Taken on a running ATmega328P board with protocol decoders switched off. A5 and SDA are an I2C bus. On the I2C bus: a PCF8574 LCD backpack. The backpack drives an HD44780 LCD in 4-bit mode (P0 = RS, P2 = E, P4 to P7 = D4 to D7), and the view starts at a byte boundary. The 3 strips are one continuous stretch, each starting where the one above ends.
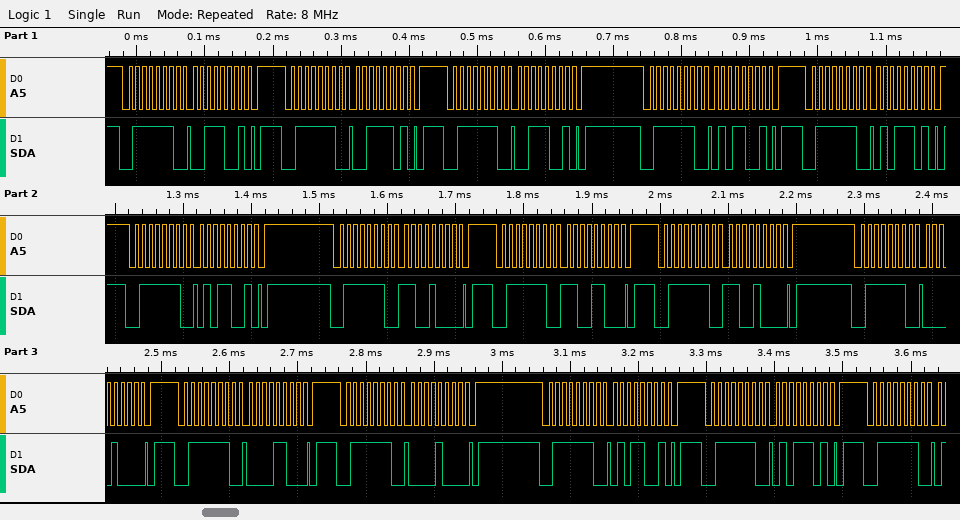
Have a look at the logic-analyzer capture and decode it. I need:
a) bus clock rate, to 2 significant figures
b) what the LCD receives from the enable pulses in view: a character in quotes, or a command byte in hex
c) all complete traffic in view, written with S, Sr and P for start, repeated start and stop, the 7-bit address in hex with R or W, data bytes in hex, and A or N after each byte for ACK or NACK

100 kHz
'5' 0xC0
S 3FW A 39 A P S 3FW A 3D A P S 3FW A 39 A P S 3FW A 59 A P S 3FW A 5D A P S 3FW A 59 A P S 3FW A C8 A P S 3FW A CC A P S 3FW A C8 A P S 3FW A 08 A P S 3FW A 0C A P S 3FW A 08 A P S 3FW A 59 A P S 3FW A 5D A P S 3FW A
